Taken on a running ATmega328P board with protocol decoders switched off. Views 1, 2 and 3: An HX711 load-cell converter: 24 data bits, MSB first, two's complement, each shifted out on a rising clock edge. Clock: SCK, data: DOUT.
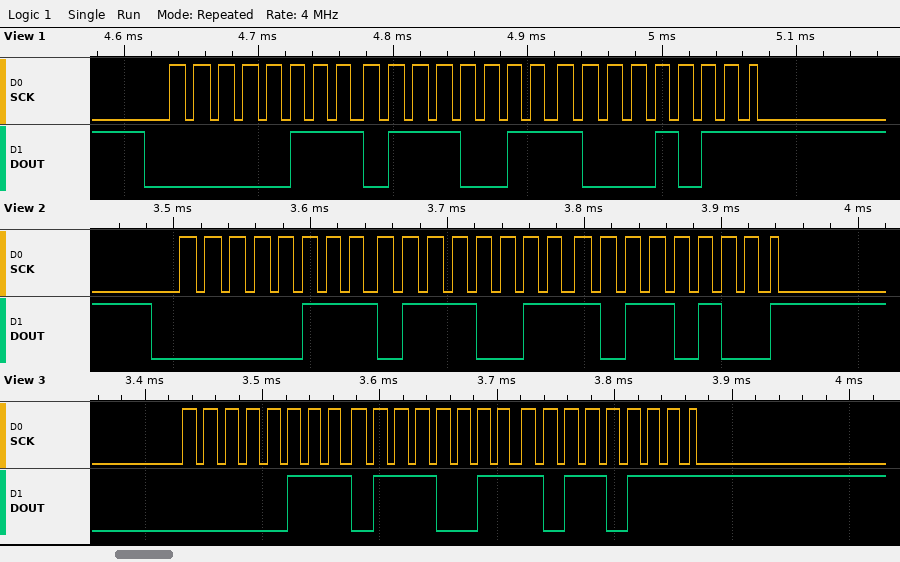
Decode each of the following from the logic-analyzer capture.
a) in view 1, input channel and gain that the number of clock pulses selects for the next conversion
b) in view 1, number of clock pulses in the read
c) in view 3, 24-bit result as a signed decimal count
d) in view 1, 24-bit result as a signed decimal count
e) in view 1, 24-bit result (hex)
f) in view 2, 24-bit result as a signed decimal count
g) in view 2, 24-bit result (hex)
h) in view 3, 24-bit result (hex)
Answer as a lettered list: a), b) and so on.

a) channel A, gain 128
b) 25
c) 488375
d) 488331
e) 0x07738B
f) 488372
g) 0x0773B4
h) 0x0773B7
